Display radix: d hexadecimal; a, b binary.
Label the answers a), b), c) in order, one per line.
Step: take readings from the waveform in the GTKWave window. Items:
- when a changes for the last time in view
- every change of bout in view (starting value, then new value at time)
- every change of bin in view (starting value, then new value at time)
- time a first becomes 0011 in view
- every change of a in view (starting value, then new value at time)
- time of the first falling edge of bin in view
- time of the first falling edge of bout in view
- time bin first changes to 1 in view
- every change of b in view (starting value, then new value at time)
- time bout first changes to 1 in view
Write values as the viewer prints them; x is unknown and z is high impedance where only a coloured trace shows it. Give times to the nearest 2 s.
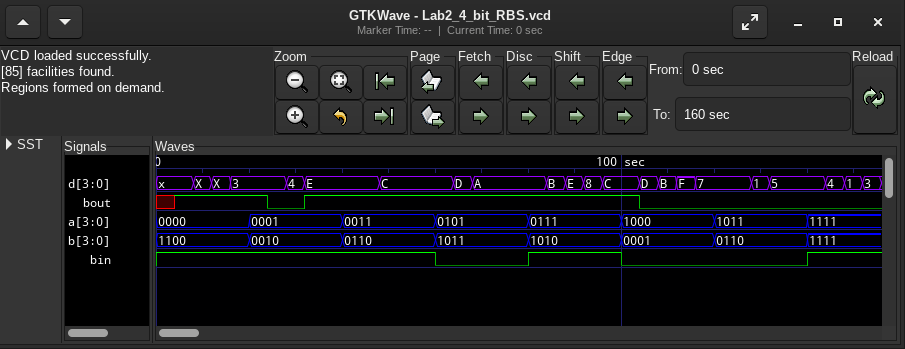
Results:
a) 140 s
b) x, 1 at 4 s, 0 at 24 s, 1 at 32 s, 0 at 104 s
c) 1, 0 at 60 s, 1 at 80 s, 0 at 100 s, 1 at 140 s
d) 40 s
e) 0000, 0001 at 20 s, 0011 at 40 s, 0101 at 60 s, 0111 at 80 s, 1000 at 100 s, 1011 at 120 s, 1111 at 140 s
f) 60 s
g) 24 s
h) 80 s
i) 1100, 0010 at 20 s, 0110 at 40 s, 1011 at 60 s, 1010 at 80 s, 0001 at 100 s, 0110 at 120 s, 1111 at 140 s
j) 4 s
